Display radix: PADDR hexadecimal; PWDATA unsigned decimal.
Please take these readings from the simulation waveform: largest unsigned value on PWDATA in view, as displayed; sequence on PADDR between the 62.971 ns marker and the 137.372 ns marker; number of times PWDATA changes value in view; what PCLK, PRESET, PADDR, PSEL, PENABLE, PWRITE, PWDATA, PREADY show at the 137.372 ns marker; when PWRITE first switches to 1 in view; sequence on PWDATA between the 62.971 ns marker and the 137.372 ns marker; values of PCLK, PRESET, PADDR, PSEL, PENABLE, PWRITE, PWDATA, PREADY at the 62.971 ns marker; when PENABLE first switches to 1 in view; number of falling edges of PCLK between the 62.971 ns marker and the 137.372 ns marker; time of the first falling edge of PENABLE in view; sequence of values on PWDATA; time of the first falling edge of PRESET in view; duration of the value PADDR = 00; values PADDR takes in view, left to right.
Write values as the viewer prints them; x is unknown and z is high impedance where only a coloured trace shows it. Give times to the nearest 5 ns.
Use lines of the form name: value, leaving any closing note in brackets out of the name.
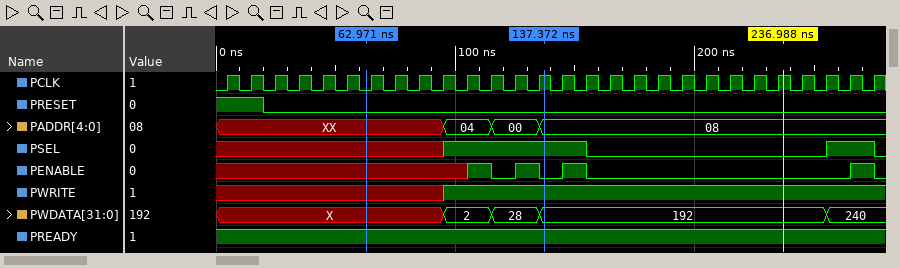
largest unsigned value on PWDATA in view, as displayed: 240
sequence on PADDR between the 62.971 ns marker and the 137.372 ns marker: XX, 04, 00, 08
number of times PWDATA changes value in view: 4
what PCLK, PRESET, PADDR, PSEL, PENABLE, PWRITE, PWDATA, PREADY show at the 137.372 ns marker: PCLK=1, PRESET=0, PADDR=08, PSEL=1, PENABLE=0, PWRITE=1, PWDATA=192, PREADY=1
when PWRITE first switches to 1 in view: 95 ns
sequence on PWDATA between the 62.971 ns marker and the 137.372 ns marker: X, 2, 28, 192
values of PCLK, PRESET, PADDR, PSEL, PENABLE, PWRITE, PWDATA, PREADY at the 62.971 ns marker: PCLK=0, PRESET=0, PADDR=XX, PSEL=x, PENABLE=x, PWRITE=x, PWDATA=X, PREADY=1
when PENABLE first switches to 1 in view: 105 ns
number of falling edges of PCLK between the 62.971 ns marker and the 137.372 ns marker: 7
time of the first falling edge of PENABLE in view: 115 ns
sequence of values on PWDATA: X, 2, 28, 192, 240
time of the first falling edge of PRESET in view: 20 ns
duration of the value PADDR = 00: 20 ns
values PADDR takes in view, left to right: XX, 04, 00, 08
